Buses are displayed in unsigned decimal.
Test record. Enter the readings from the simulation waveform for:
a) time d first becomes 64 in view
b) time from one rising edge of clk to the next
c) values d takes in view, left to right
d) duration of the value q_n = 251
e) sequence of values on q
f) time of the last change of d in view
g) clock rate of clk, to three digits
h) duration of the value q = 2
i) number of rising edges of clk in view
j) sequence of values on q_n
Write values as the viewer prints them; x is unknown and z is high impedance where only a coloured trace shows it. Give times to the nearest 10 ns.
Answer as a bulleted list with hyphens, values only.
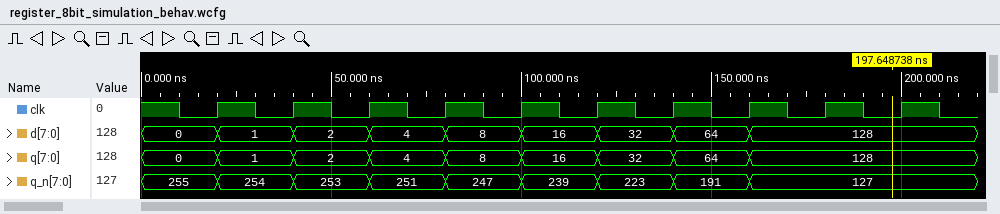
- 140 ns
- 20 ns
- 0, 1, 2, 4, 8, 16, 32, 64, 128
- 20 ns
- 0, 1, 2, 4, 8, 16, 32, 64, 128
- 160 ns
- 50.0 MHz
- 20 ns
- 10
- 255, 254, 253, 251, 247, 239, 223, 191, 127
